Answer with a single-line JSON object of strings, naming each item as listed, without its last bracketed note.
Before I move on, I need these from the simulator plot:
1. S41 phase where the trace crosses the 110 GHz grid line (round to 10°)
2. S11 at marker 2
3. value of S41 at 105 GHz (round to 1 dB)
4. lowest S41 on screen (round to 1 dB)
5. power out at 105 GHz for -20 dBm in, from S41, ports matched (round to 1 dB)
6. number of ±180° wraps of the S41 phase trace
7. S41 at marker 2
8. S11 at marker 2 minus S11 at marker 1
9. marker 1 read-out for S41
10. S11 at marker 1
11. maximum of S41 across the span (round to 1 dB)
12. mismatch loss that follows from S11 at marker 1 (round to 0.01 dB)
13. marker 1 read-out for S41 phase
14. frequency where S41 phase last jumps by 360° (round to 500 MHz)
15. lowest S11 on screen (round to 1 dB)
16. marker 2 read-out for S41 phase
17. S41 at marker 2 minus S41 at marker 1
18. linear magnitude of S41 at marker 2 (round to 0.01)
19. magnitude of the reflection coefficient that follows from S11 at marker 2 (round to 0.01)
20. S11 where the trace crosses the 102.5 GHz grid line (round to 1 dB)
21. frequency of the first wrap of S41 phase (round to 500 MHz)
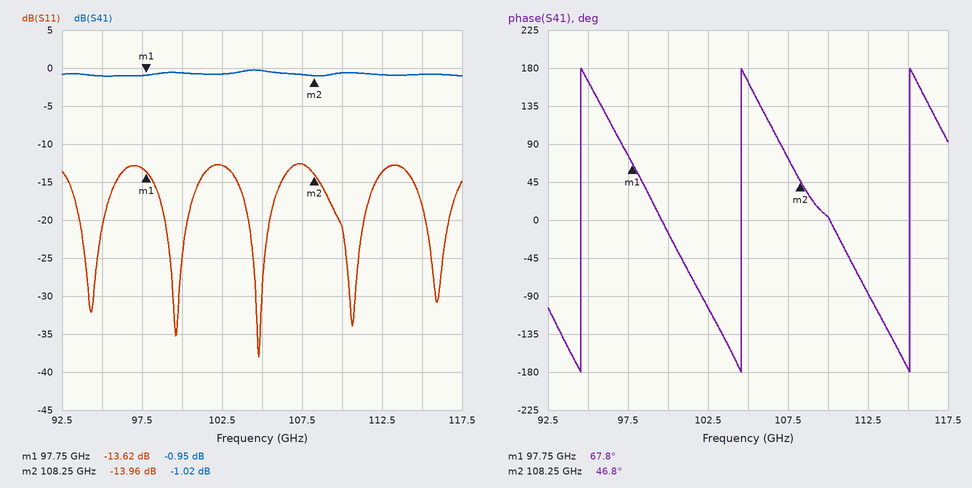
{"S41 phase where the trace crosses the 110 GHz grid line": "0°", "S11 at marker 2": "-13.96 dB", "value of S41 at 105 GHz": "0 dB", "lowest S41 on screen": "-1 dB", "power out at 105 GHz for -20 dBm in, from S41, ports matched": "-20 dBm", "number of ±180° wraps of the S41 phase trace": "3", "S41 at marker 2": "-1.02 dB", "S11 at marker 2 minus S11 at marker 1": "-0.34 dB", "marker 1 read-out for S41": "-0.95 dB", "S11 at marker 1": "-13.62 dB", "maximum of S41 across the span": "0 dB", "mismatch loss that follows from S11 at marker 1": "0.19 dB", "marker 1 read-out for S41 phase": "67.8°", "frequency where S41 phase last jumps by 360°": "115.0 GHz", "lowest S11 on screen": "-38 dB", "marker 2 read-out for S41 phase": "46.8°", "S41 at marker 2 minus S41 at marker 1": "-0.07 dB", "linear magnitude of S41 at marker 2": "0.89", "magnitude of the reflection coefficient that follows from S11 at marker 2": "0.20", "S11 where the trace crosses the 102.5 GHz grid line": "-13 dB", "frequency of the first wrap of S41 phase": "94.5 GHz"}
